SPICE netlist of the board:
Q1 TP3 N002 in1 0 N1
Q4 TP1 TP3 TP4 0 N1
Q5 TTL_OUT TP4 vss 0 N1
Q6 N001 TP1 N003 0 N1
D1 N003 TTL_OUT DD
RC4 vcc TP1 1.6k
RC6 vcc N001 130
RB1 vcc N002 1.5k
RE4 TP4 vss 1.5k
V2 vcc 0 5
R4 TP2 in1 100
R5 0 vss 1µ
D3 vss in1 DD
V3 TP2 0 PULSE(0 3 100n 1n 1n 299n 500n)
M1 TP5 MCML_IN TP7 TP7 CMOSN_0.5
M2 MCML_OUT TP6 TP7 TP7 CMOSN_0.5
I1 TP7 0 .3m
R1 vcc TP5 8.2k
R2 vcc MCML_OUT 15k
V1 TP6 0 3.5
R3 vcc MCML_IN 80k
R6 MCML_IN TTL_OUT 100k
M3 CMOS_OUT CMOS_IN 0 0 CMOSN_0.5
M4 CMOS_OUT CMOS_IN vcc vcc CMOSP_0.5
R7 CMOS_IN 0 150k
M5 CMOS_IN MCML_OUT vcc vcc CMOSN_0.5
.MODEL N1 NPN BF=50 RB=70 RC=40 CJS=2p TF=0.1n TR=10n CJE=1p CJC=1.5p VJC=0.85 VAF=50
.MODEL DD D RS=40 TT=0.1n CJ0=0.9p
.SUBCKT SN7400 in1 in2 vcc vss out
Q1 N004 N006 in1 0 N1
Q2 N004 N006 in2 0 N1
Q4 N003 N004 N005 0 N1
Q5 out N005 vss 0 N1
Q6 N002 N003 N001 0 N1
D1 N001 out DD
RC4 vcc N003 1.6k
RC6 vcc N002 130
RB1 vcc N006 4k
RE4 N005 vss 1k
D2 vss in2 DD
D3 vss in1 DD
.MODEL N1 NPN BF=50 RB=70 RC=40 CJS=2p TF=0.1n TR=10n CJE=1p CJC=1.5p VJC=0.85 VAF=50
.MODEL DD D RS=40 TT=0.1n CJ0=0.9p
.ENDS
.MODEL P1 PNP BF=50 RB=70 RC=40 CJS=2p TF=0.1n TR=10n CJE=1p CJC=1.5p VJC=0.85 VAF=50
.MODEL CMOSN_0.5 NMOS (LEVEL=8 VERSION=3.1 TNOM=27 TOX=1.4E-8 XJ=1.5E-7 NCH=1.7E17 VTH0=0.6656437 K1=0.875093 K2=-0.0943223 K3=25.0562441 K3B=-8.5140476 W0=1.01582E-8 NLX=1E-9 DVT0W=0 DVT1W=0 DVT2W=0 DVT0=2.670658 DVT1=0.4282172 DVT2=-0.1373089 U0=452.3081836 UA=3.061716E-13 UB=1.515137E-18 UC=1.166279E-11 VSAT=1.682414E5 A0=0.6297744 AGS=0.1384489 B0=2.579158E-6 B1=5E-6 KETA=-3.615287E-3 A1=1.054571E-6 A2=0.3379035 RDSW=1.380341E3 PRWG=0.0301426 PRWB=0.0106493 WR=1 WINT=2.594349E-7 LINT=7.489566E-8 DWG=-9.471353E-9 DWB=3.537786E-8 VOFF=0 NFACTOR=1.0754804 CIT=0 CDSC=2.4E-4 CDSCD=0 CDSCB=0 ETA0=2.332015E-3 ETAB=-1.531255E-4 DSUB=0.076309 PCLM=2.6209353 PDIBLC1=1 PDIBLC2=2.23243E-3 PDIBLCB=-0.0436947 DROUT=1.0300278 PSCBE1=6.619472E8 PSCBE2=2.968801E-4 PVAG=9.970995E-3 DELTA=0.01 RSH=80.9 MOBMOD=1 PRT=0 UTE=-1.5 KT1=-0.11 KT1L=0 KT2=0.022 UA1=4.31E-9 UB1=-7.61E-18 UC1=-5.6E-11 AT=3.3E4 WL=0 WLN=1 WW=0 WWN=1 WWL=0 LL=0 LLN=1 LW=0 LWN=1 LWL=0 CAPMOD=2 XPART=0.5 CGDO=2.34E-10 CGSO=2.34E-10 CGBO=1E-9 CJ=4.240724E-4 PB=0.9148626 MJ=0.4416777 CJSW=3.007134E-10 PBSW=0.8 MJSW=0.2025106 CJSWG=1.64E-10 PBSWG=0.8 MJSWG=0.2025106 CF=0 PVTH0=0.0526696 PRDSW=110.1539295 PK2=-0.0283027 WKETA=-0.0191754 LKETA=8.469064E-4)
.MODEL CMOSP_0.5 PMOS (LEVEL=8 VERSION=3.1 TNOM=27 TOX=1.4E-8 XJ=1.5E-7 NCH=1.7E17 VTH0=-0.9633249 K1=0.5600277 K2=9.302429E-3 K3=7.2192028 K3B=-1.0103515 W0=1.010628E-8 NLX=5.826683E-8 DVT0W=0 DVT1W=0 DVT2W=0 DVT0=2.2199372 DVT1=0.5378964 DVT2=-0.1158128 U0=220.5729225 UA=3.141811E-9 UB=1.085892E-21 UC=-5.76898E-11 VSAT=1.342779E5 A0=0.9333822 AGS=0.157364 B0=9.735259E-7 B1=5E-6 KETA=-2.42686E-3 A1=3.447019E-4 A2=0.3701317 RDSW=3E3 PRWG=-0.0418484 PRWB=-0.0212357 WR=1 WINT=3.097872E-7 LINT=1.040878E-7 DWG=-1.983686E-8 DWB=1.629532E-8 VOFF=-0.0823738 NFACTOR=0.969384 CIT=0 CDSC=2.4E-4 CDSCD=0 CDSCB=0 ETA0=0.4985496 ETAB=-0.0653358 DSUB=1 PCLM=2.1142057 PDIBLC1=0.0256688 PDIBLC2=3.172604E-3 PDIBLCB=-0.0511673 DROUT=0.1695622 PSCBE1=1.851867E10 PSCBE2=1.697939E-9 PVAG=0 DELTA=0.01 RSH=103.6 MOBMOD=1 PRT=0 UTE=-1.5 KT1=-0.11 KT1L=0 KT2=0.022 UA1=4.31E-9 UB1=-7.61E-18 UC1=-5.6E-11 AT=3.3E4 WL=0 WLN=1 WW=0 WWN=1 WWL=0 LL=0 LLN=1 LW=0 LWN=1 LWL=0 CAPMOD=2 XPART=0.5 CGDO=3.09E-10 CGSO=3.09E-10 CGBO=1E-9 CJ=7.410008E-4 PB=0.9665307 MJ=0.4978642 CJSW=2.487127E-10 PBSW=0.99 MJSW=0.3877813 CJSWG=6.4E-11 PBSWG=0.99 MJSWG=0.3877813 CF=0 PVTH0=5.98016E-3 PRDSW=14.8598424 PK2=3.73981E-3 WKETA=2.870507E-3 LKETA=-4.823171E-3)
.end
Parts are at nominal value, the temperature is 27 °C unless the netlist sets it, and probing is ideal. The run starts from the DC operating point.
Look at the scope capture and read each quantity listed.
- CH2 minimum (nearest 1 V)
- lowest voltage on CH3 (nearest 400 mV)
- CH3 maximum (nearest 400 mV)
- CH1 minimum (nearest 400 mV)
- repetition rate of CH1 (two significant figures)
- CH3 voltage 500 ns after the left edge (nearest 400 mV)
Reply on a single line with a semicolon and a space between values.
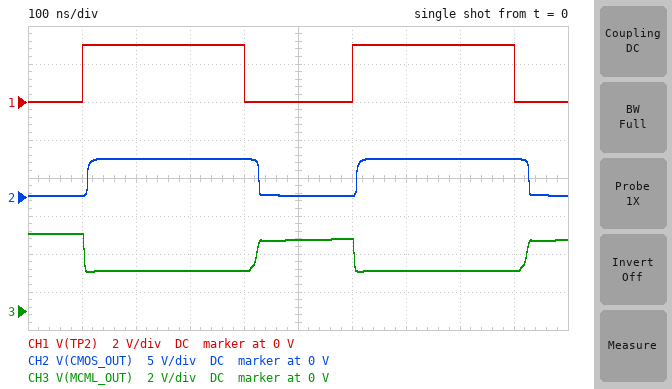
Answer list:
0 V; 2.0 V; 4.0 V; 0 V; 2.0 MHz; 3.6 V
